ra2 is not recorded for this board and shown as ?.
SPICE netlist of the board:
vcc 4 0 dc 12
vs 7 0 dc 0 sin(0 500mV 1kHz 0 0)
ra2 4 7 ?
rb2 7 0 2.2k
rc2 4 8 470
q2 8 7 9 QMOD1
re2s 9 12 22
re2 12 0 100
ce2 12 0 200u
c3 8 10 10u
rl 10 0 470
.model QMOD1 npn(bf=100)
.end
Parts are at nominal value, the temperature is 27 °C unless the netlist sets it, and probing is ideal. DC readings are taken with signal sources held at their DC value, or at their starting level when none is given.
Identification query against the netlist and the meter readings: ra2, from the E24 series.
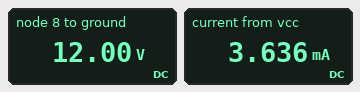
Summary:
3.3 kΩ
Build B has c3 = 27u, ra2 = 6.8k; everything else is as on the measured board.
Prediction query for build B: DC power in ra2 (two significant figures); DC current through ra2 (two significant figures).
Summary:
21 mW
1.8 mA
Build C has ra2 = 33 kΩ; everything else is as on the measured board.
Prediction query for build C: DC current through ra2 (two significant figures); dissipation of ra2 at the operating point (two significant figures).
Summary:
360 µA
4.4 mW
